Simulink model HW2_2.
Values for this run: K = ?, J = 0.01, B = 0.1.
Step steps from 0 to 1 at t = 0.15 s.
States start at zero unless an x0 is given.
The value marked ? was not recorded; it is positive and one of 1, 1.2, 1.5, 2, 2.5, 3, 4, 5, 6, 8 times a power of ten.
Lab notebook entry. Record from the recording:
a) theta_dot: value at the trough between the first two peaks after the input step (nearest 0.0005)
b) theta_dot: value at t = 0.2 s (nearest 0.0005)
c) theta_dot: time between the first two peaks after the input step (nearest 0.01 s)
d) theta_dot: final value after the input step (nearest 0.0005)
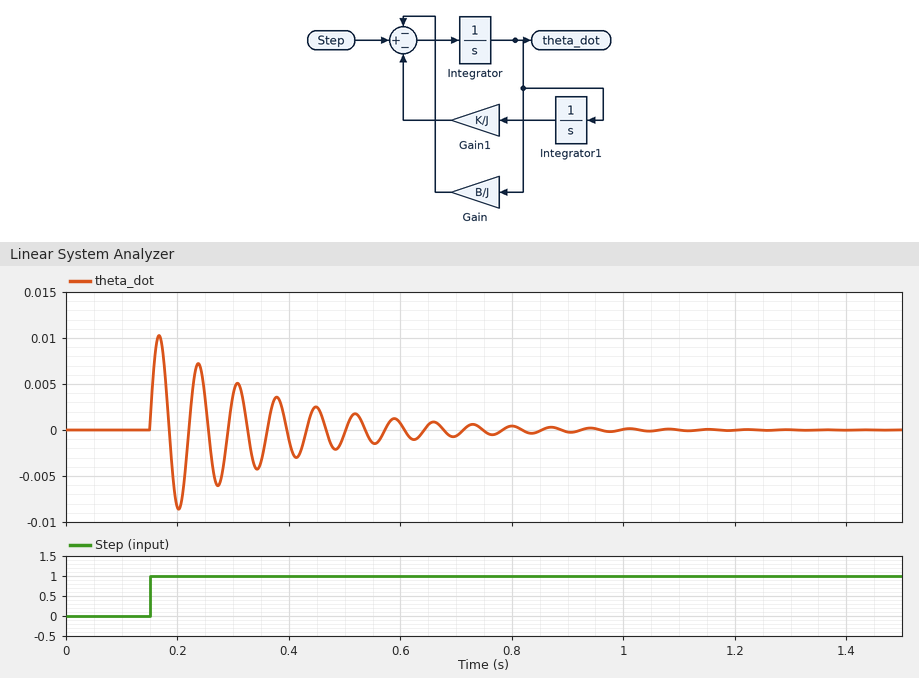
-0.0085
-0.0085
0.07 s
0.0000
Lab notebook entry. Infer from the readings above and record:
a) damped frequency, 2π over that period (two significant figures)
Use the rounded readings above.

90 rad/s
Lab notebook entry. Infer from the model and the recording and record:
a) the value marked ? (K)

80
